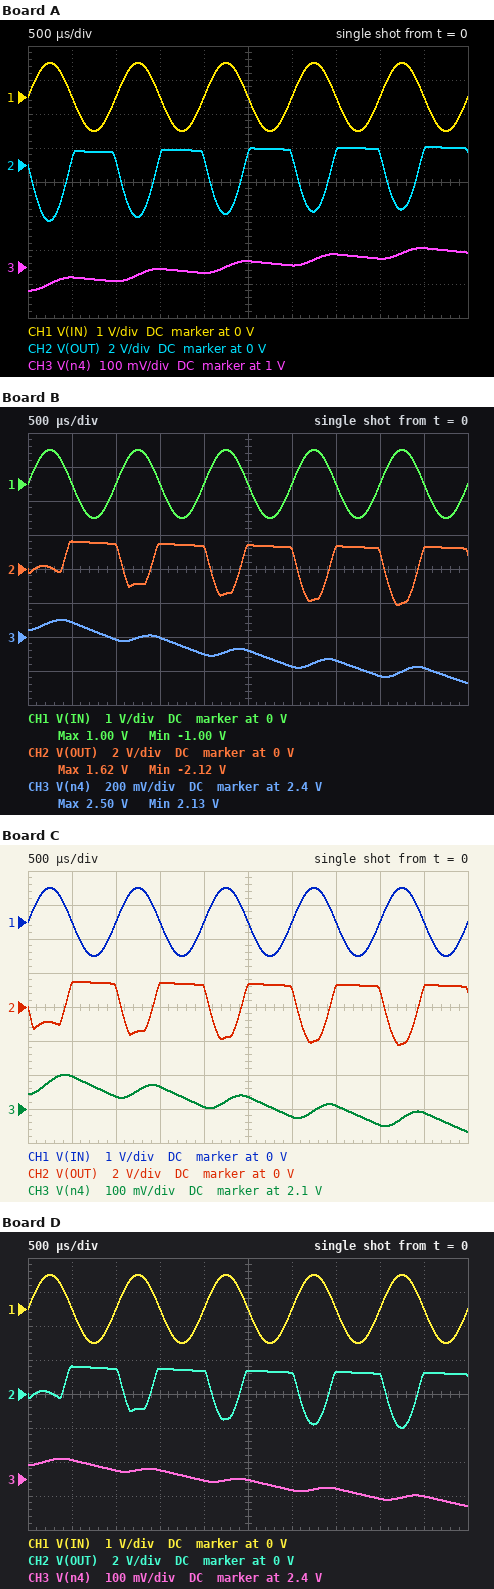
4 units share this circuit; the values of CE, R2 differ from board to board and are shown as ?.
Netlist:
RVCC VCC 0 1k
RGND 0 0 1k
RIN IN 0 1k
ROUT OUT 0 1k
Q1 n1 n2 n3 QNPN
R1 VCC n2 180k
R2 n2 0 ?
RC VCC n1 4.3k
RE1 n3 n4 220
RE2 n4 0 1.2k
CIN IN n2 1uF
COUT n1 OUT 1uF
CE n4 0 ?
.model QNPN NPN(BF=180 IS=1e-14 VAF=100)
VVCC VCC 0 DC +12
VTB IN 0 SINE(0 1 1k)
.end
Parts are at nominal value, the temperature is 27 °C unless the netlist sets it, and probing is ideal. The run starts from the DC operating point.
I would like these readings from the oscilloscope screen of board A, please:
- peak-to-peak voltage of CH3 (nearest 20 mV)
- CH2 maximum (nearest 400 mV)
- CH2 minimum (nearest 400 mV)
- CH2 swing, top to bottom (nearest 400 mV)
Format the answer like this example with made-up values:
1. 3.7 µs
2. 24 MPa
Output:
1. 120 mV
2. 1.2 V
3. -3.2 V
4. 4.4 V
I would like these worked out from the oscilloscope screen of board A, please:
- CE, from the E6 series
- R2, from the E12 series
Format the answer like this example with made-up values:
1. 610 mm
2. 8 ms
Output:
1. 33 µF
2. 33 kΩ
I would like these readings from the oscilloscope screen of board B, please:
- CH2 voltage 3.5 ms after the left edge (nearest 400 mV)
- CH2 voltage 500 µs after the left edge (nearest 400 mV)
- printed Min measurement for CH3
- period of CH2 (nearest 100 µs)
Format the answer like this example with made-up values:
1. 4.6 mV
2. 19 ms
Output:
1. 1.2 V
2. 1.6 V
3. 2.13 V
4. 1.0 ms
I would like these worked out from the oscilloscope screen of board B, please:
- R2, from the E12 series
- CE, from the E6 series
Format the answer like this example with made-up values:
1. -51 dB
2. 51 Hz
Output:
1. 100 kΩ
2. 10 µF
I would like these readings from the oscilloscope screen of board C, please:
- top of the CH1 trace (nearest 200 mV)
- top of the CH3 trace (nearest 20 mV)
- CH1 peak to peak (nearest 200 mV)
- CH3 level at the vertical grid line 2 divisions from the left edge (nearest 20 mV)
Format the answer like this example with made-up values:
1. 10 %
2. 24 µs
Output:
1. 1.0 V
2. 2.20 V
3. 2.0 V
4. 2.14 V
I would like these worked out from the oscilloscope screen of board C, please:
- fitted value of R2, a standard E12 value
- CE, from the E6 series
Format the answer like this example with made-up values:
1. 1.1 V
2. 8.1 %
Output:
1. 82 kΩ
2. 15 µF
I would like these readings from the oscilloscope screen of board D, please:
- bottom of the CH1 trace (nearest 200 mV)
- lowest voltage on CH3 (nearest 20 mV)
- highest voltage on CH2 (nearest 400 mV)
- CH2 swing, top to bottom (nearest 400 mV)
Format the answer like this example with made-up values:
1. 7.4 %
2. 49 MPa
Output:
1. -1.0 V
2. 2.32 V
3. 1.6 V
4. 3.6 V
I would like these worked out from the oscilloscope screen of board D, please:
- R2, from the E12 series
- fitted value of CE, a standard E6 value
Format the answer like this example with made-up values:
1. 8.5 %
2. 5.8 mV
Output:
1. 100 kΩ
2. 33 µF
